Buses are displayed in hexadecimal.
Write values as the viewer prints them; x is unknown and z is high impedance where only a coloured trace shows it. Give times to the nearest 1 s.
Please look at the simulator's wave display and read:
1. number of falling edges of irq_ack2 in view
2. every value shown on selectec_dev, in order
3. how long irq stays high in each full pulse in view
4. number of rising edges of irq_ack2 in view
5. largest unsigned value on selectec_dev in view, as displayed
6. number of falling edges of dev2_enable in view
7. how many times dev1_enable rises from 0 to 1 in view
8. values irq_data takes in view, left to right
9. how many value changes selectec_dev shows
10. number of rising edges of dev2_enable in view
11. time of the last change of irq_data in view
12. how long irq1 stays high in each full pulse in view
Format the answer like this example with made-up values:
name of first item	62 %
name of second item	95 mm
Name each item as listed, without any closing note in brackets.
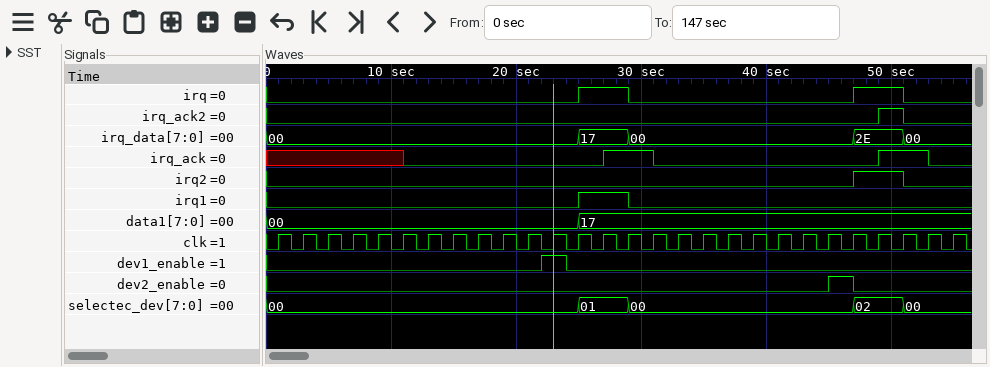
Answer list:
number of falling edges of irq_ack2 in view	1
every value shown on selectec_dev, in order	00, 01, 00, 02, 00
how long irq stays high in each full pulse in view	4 s, 4 s
number of rising edges of irq_ack2 in view	1
largest unsigned value on selectec_dev in view, as displayed	02
number of falling edges of dev2_enable in view	1
how many times dev1_enable rises from 0 to 1 in view	1
values irq_data takes in view, left to right	00, 17, 00, 2E, 00
how many value changes selectec_dev shows	4
number of rising edges of dev2_enable in view	1
time of the last change of irq_data in view	51 s
how long irq1 stays high in each full pulse in view	4 s
